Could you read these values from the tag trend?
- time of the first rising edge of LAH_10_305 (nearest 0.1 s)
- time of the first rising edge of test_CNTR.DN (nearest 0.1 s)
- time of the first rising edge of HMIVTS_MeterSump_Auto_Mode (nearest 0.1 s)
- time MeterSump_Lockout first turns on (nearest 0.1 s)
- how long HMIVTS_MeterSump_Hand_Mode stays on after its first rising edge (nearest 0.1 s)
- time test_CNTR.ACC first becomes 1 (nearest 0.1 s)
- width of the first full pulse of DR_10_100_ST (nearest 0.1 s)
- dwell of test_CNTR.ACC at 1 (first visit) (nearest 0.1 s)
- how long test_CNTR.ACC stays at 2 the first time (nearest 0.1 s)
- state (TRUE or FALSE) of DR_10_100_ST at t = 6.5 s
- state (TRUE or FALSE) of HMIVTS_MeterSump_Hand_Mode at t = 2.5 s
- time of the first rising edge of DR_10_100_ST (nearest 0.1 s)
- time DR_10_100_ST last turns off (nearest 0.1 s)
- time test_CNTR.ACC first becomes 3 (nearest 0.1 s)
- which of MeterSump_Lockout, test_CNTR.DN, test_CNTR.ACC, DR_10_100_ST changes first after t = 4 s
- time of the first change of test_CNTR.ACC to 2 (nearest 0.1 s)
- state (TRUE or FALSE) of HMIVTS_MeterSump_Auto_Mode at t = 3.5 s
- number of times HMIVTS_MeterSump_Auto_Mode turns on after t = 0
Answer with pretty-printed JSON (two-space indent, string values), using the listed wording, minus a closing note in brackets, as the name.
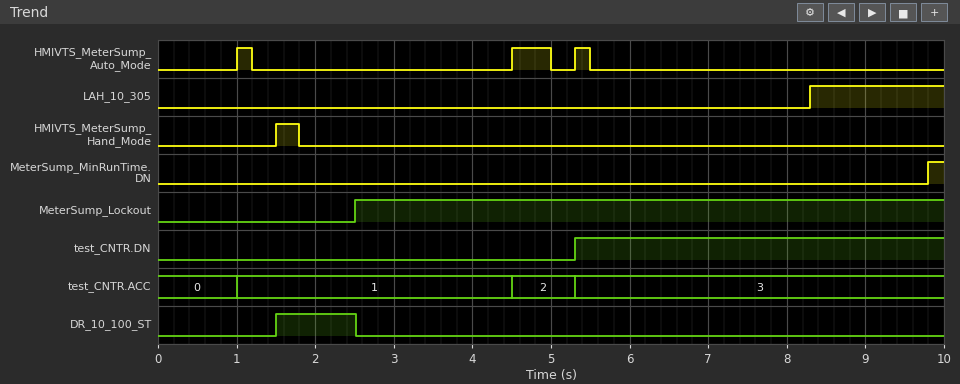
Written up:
{
  "time of the first rising edge of LAH_10_305": "8.3 s",
  "time of the first rising edge of test_CNTR.DN": "5.3 s",
  "time of the first rising edge of HMIVTS_MeterSump_Auto_Mode": "1.0 s",
  "time MeterSump_Lockout first turns on": "2.5 s",
  "how long HMIVTS_MeterSump_Hand_Mode stays on after its first rising edge": "0.3 s",
  "time test_CNTR.ACC first becomes 1": "1.0 s",
  "width of the first full pulse of DR_10_100_ST": "1.0 s",
  "dwell of test_CNTR.ACC at 1 (first visit)": "3.5 s",
  "how long test_CNTR.ACC stays at 2 the first time": "0.8 s",
  "state (TRUE or FALSE) of DR_10_100_ST at t = 6.5 s": "FALSE",
  "state (TRUE or FALSE) of HMIVTS_MeterSump_Hand_Mode at t = 2.5 s": "FALSE",
  "time of the first rising edge of DR_10_100_ST": "1.5 s",
  "time DR_10_100_ST last turns off": "2.5 s",
  "time test_CNTR.ACC first becomes 3": "5.3 s",
  "which of MeterSump_Lockout, test_CNTR.DN, test_CNTR.ACC, DR_10_100_ST changes first after t = 4 s": "test_CNTR.ACC",
  "time of the first change of test_CNTR.ACC to 2": "4.5 s",
  "state (TRUE or FALSE) of HMIVTS_MeterSump_Auto_Mode at t = 3.5 s": "FALSE",
  "number of times HMIVTS_MeterSump_Auto_Mode turns on after t = 0": "3"
}
